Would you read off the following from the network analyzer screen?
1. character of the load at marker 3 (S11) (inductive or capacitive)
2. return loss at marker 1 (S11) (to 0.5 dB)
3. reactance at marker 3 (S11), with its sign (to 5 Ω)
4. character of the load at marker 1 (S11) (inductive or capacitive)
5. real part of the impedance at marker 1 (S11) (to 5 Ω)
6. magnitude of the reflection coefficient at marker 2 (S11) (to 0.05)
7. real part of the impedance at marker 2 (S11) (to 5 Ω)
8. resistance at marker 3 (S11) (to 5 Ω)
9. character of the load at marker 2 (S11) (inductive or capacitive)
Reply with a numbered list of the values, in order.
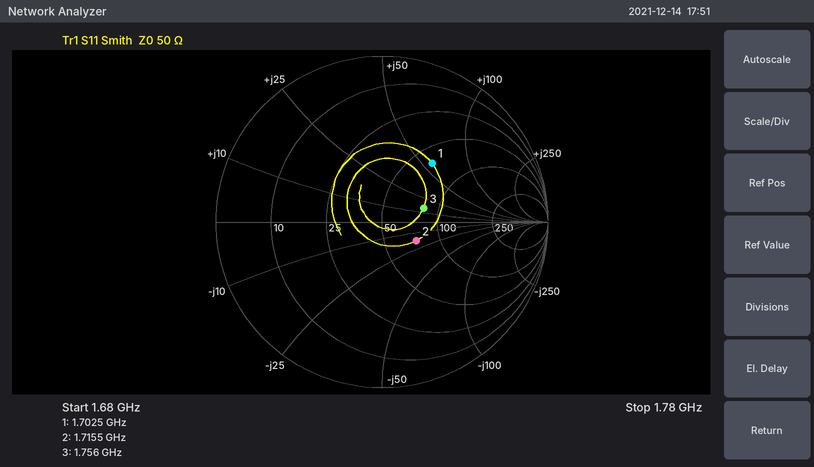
1. inductive
2. 6.5 dB
3. +15 Ω
4. inductive
5. 65 Ω
6. 0.25
7. 75 Ω
8. 80 Ω
9. capacitive
